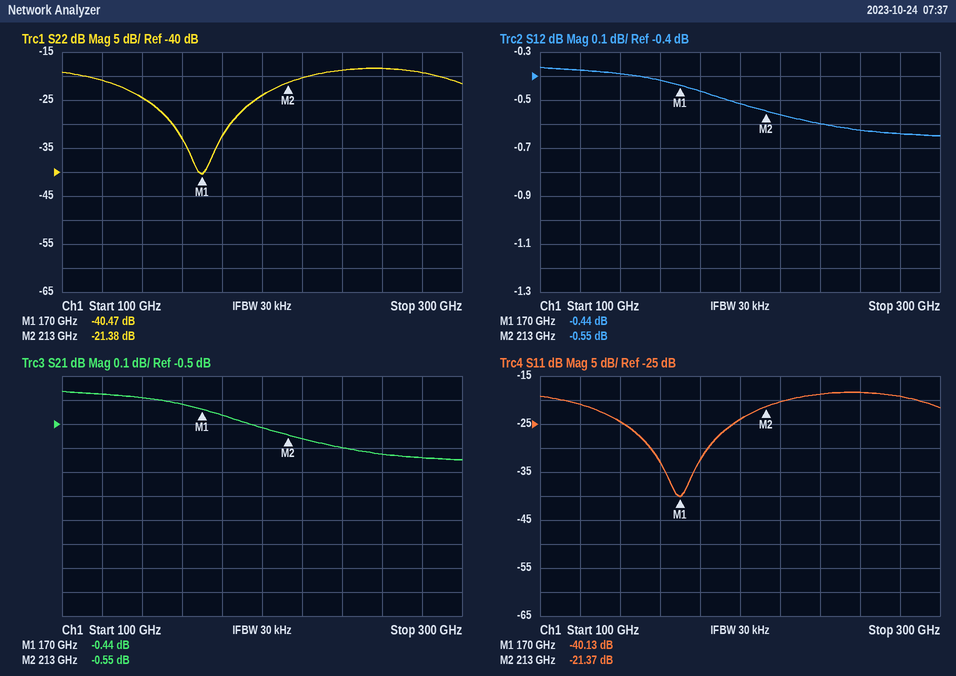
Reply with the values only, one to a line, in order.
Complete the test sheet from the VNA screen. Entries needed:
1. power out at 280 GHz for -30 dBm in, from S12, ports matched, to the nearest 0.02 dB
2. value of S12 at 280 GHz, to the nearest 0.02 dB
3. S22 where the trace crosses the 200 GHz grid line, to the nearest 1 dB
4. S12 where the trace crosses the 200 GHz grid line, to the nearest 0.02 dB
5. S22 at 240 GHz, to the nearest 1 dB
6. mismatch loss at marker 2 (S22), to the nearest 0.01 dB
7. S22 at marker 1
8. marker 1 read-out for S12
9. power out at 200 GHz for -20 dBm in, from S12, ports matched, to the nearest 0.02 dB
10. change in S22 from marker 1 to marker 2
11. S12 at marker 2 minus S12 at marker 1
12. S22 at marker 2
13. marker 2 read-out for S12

-30.64 dBm
-0.64 dB
-24 dB
-0.52 dB
-19 dB
0.03 dB
-40.47 dB
-0.44 dB
-20.52 dBm
19.09 dB
-0.11 dB
-21.38 dB
-0.55 dB
